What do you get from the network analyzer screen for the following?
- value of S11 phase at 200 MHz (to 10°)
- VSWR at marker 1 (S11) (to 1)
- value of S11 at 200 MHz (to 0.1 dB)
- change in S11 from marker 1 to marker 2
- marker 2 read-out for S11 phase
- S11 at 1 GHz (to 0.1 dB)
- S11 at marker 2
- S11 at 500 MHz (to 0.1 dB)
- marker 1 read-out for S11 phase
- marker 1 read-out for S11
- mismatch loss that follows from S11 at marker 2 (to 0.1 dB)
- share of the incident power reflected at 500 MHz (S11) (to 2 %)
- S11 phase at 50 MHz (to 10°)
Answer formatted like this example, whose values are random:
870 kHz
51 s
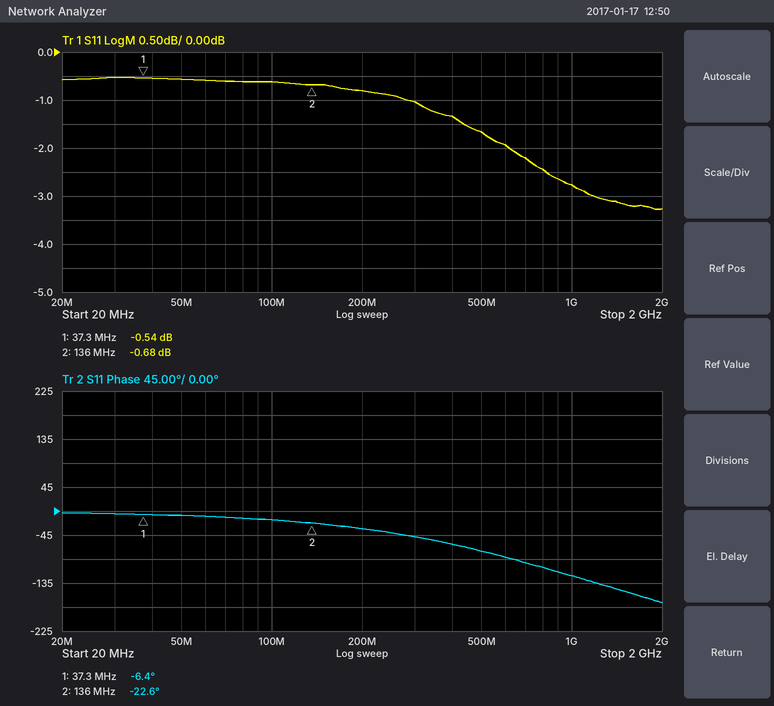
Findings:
-30°
32
-0.8 dB
-0.14 dB
-22.6°
-2.8 dB
-0.68 dB
-1.7 dB
-6.4°
-0.54 dB
8.4 dB
68 %
-10°
